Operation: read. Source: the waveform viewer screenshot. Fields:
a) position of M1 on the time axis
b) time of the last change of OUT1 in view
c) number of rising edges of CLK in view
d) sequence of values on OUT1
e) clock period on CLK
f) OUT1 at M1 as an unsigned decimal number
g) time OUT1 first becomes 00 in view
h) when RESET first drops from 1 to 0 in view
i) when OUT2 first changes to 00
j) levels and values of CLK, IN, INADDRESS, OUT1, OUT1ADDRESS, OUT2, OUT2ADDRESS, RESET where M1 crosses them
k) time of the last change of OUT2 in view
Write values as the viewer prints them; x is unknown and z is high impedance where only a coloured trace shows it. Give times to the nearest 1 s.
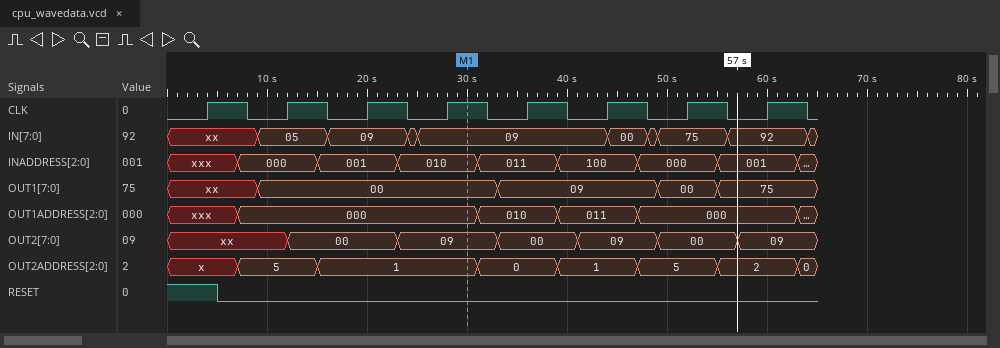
30 s
55 s
8
xx, 00, 09, 00, 75
8 s
0
9 s
5 s
12 s
CLK=1, IN=09, INADDRESS=010, OUT1=00, OUT1ADDRESS=000, OUT2=09, OUT2ADDRESS=1, RESET=0
57 s
